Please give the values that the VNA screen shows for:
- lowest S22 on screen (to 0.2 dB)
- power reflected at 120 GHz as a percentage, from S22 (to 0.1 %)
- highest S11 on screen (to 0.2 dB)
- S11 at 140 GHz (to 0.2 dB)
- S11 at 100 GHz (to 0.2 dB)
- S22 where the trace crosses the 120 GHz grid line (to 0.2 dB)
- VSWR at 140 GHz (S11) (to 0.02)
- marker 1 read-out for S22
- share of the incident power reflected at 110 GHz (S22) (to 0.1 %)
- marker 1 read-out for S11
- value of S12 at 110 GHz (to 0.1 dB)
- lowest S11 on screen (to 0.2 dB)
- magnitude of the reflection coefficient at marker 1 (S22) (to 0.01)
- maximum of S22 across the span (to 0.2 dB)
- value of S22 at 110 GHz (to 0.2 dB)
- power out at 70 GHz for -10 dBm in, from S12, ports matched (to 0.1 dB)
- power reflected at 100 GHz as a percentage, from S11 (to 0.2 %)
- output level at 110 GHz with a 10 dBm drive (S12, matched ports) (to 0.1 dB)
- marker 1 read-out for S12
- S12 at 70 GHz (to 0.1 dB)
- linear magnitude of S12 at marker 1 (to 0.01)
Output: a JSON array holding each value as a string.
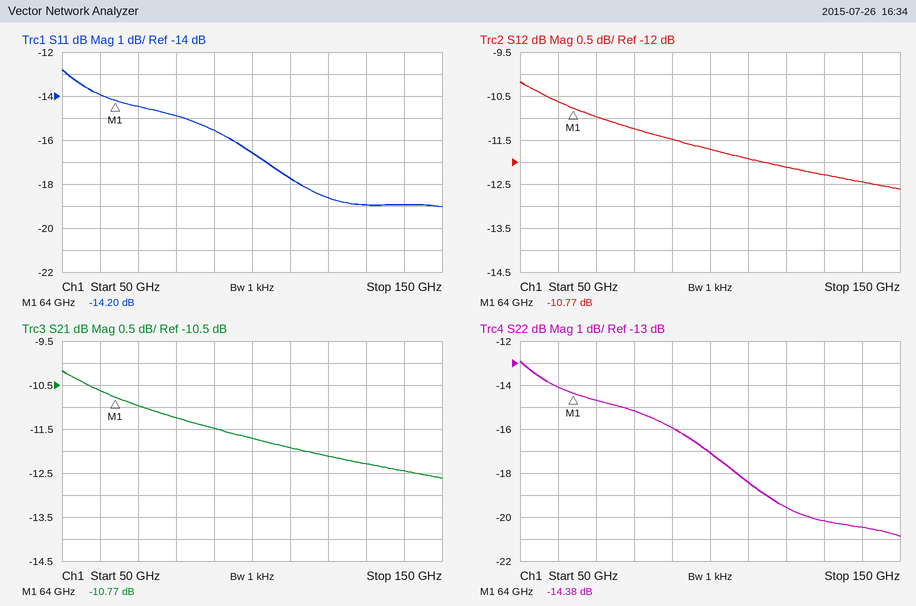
["-20.8 dB", "1.1 %", "-12.8 dB", "-19.0 dB", "-16.6 dB", "-19.6 dB", "1.26", "-14.38 dB", "1.4 %", "-14.20 dB", "-11.9 dB", "-19.0 dB", "0.19", "-13.0 dB", "-18.4 dB", "-21.0 dBm", "2.2 %", "-1.9 dBm", "-10.77 dB", "-11.0 dB", "0.29"]
